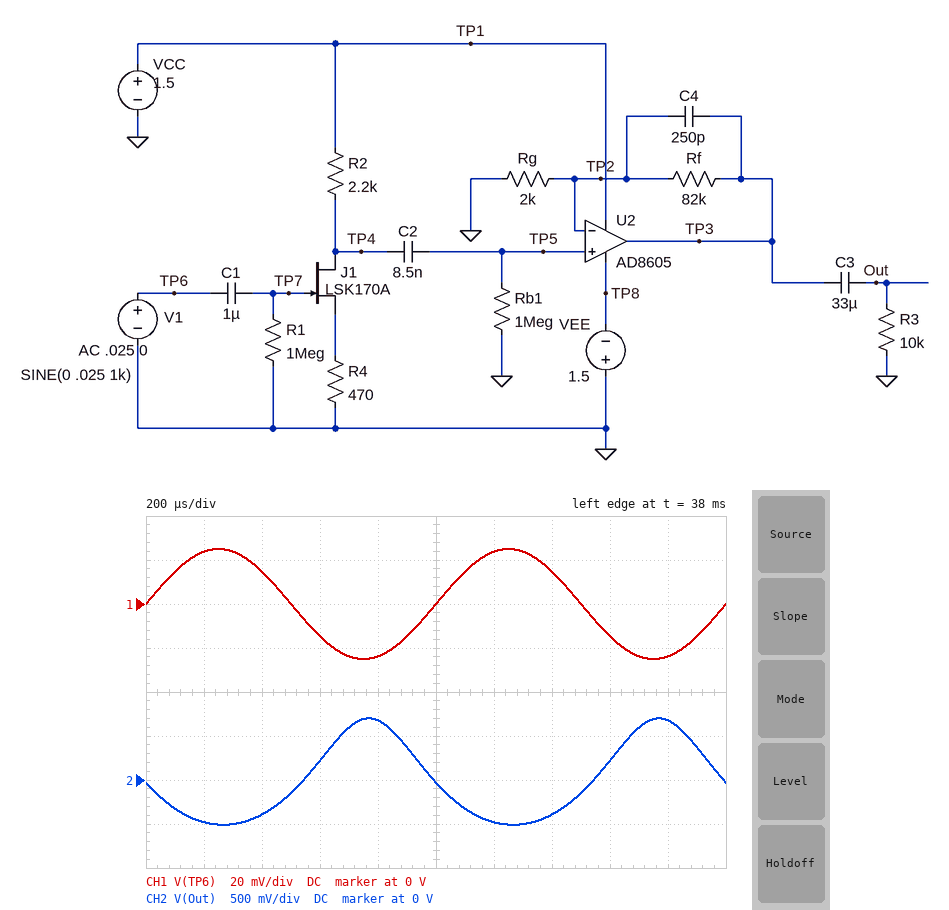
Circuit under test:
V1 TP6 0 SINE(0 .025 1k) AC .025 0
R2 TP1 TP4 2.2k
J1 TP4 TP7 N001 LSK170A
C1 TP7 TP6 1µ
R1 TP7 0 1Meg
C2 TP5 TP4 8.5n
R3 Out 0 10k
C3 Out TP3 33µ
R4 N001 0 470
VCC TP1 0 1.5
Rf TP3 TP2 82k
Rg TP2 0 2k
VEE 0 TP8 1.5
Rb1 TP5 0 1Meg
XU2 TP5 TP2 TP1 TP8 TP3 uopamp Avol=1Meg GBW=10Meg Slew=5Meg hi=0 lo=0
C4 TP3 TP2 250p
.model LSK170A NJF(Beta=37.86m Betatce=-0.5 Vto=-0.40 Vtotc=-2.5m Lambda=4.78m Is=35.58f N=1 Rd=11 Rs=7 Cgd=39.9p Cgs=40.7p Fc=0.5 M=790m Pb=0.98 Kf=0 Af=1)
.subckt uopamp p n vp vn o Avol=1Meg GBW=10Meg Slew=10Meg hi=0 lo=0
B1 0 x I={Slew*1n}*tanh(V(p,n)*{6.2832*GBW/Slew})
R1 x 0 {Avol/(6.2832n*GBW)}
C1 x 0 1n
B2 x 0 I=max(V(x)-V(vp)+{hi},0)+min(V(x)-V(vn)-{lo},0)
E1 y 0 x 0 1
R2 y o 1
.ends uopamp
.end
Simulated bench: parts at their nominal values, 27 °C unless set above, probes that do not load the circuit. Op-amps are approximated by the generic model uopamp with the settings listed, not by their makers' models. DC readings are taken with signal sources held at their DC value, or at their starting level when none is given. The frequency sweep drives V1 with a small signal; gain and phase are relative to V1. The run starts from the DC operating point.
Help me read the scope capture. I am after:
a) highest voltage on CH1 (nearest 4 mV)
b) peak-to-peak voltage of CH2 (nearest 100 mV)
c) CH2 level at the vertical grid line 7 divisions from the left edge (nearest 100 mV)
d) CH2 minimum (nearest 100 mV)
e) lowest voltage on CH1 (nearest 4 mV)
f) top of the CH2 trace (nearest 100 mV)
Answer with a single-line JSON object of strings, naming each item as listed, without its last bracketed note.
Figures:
{"highest voltage on CH1": "24 mV", "peak-to-peak voltage of CH2": "1.2 V", "CH2 level at the vertical grid line 7 divisions from the left edge": "-400 mV", "CH2 minimum": "-500 mV", "lowest voltage on CH1": "-24 mV", "top of the CH2 trace": "700 mV"}
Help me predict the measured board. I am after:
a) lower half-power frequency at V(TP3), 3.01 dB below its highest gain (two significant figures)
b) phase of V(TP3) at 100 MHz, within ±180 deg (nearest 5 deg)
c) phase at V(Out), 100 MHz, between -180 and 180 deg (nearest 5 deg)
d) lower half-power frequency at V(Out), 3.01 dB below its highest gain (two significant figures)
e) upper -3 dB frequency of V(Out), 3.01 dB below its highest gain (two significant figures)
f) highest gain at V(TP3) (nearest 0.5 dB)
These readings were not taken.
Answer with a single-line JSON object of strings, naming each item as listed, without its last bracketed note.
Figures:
{"lower half-power frequency at V(TP3), 3.01 dB below its highest gain": "19 Hz", "phase of V(TP3) at 100 MHz, within ±180 deg": "-80 deg", "phase at V(Out), 100 MHz, between -180 and 180 deg": "-80 deg", "lower half-power frequency at V(Out), 3.01 dB below its highest gain": "19 Hz", "upper -3 dB frequency of V(Out), 3.01 dB below its highest gain": "7.6 kHz", "highest gain at V(TP3)": "26.5 dB"}
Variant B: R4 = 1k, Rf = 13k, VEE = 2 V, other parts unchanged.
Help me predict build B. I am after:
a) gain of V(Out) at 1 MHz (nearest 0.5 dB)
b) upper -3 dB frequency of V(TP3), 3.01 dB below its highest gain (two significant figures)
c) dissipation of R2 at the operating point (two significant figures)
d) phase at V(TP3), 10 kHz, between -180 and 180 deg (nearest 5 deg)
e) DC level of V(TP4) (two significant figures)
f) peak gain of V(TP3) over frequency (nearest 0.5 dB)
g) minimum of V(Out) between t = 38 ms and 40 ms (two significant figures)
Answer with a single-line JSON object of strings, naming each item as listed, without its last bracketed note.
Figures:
{"gain of V(Out) at 1 MHz": "5.5 dB", "upper -3 dB frequency of V(TP3), 3.01 dB below its highest gain": "48 kHz", "dissipation of R2 at the operating point": "210 µW", "phase at V(TP3), 10 kHz, between -180 and 180 deg": "170 deg", "DC level of V(TP4)": "820 mV", "peak gain of V(TP3) over frequency": "23.0 dB", "minimum of V(Out) between t = 38 ms and 40 ms": "-360 mV"}
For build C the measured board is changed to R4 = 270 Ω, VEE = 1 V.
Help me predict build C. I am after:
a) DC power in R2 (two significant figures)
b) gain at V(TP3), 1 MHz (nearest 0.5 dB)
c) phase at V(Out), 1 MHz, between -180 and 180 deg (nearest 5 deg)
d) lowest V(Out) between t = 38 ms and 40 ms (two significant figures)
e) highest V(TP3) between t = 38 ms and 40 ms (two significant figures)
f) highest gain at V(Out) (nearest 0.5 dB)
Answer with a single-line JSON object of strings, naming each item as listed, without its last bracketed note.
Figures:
{"DC power in R2": "760 µW", "gain at V(TP3), 1 MHz": "-14.0 dB", "phase at V(Out), 1 MHz, between -180 and 180 deg": "110 deg", "lowest V(Out) between t = 38 ms and 40 ms": "-150 mV", "highest V(TP3) between t = 38 ms and 40 ms": "170 mV", "highest gain at V(Out)": "16.0 dB"}
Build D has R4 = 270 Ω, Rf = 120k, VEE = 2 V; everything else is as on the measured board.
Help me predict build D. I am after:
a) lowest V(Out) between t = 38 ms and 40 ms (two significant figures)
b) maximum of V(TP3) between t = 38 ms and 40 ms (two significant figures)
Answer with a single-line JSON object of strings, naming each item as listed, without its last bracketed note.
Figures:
{"lowest V(Out) between t = 38 ms and 40 ms": "-210 mV", "maximum of V(TP3) between t = 38 ms and 40 ms": "240 mV"}
